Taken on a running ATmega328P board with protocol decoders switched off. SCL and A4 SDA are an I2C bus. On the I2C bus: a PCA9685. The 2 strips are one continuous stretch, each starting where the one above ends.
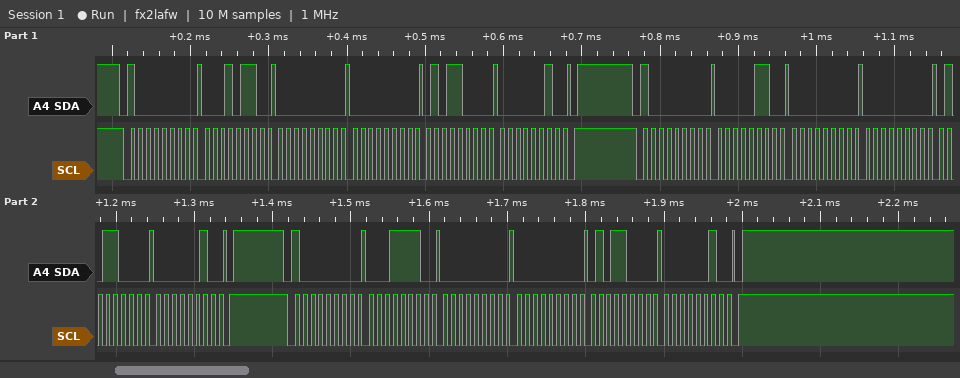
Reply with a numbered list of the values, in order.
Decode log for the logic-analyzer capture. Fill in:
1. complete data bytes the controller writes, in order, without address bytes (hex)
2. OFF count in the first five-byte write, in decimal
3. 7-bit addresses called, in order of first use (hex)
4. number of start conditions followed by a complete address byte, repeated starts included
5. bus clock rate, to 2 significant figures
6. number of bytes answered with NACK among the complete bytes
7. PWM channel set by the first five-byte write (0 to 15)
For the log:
1. 16 00 00 58 02 06 00 00 58 02 1E 00 00 58 02
2. 600
3. 0x40
4. 3
5. 100 kHz
6. 0
7. 4
